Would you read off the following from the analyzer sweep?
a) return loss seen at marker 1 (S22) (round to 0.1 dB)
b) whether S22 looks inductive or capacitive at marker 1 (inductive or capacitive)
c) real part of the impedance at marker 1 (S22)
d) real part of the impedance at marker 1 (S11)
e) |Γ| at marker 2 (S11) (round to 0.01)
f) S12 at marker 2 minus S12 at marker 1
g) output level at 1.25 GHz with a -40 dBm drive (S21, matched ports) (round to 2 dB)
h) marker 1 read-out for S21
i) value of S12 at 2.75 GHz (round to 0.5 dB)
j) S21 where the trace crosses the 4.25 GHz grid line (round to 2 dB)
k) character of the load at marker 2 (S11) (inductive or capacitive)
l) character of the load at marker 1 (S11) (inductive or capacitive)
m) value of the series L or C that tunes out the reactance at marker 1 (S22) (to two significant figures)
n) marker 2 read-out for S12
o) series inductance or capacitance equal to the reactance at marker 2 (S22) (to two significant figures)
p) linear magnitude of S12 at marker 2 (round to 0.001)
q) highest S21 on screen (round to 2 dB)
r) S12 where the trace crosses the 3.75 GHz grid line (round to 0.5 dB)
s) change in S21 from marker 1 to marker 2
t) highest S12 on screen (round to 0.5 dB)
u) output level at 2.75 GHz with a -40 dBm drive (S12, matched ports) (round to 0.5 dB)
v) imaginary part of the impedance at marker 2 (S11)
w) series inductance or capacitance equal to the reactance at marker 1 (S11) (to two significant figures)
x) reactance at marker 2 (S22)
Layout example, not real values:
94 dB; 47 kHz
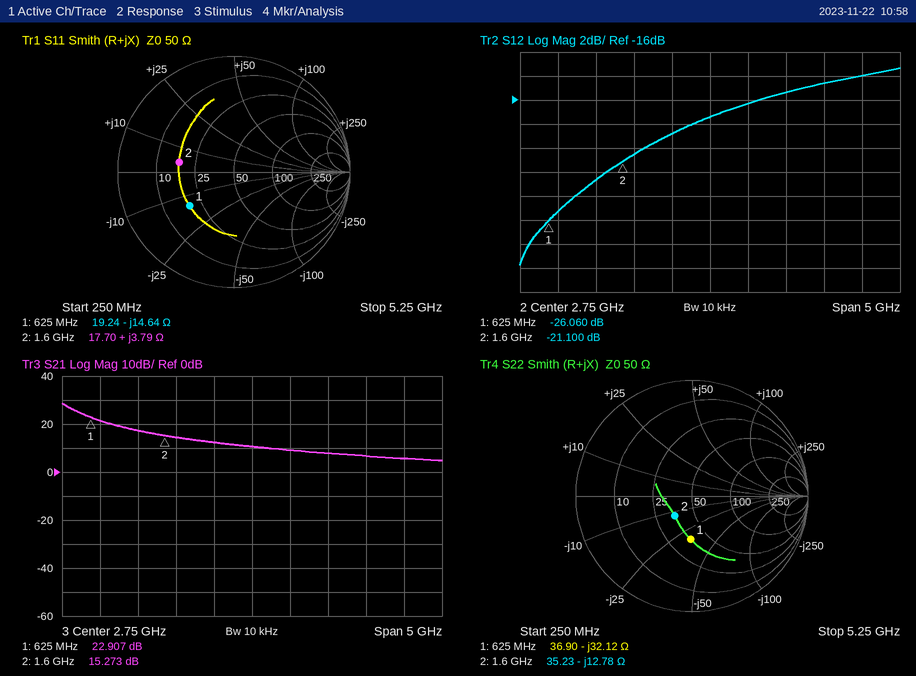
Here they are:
8.5 dB; capacitive; 36.90 Ω; 19.24 Ω; 0.48; 4.960 dB; -22 dBm; 22.907 dB; -17.5 dB; 6 dB; inductive; capacitive; 8.2 nH; -21.100 dB; 7.8 pF; 0.088; 28 dB; -15.5 dB; -7.634 dB; -13.5 dB; -57.5 dBm; +3.79 Ω; 17 pF; -12.78 Ω
